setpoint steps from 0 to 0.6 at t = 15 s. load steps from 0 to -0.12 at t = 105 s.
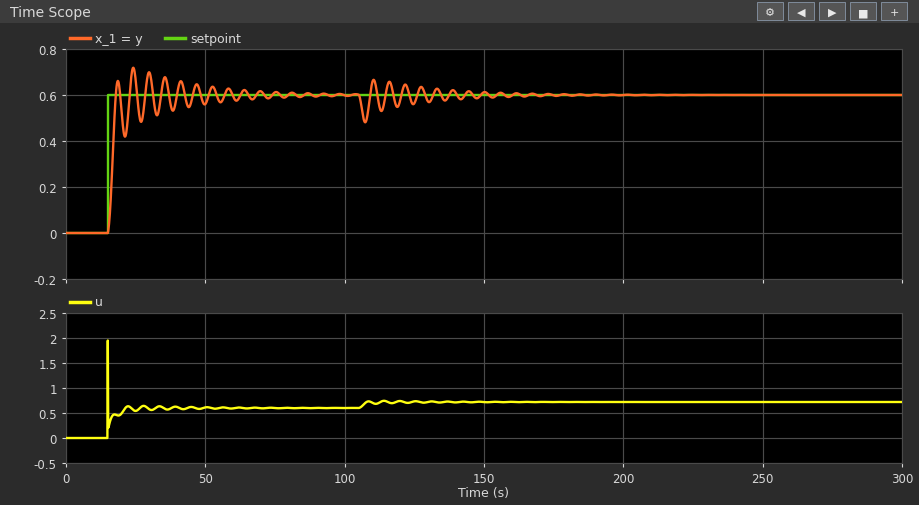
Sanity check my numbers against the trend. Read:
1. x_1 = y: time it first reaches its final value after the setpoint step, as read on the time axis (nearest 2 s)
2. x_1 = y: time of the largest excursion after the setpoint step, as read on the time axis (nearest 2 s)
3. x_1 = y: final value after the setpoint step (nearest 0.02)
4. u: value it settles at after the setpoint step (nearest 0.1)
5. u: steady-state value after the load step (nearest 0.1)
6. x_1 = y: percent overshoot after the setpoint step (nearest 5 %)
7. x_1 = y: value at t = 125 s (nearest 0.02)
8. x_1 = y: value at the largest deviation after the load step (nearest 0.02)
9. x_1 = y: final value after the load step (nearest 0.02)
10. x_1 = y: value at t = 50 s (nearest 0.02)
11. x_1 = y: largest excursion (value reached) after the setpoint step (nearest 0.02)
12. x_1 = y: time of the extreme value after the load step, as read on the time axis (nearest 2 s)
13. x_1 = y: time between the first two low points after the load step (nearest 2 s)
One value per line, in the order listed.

18 s
24 s
0.60
0.6
0.7
20 %
0.56
0.48
0.60
0.56
0.72
108 s
6 s
